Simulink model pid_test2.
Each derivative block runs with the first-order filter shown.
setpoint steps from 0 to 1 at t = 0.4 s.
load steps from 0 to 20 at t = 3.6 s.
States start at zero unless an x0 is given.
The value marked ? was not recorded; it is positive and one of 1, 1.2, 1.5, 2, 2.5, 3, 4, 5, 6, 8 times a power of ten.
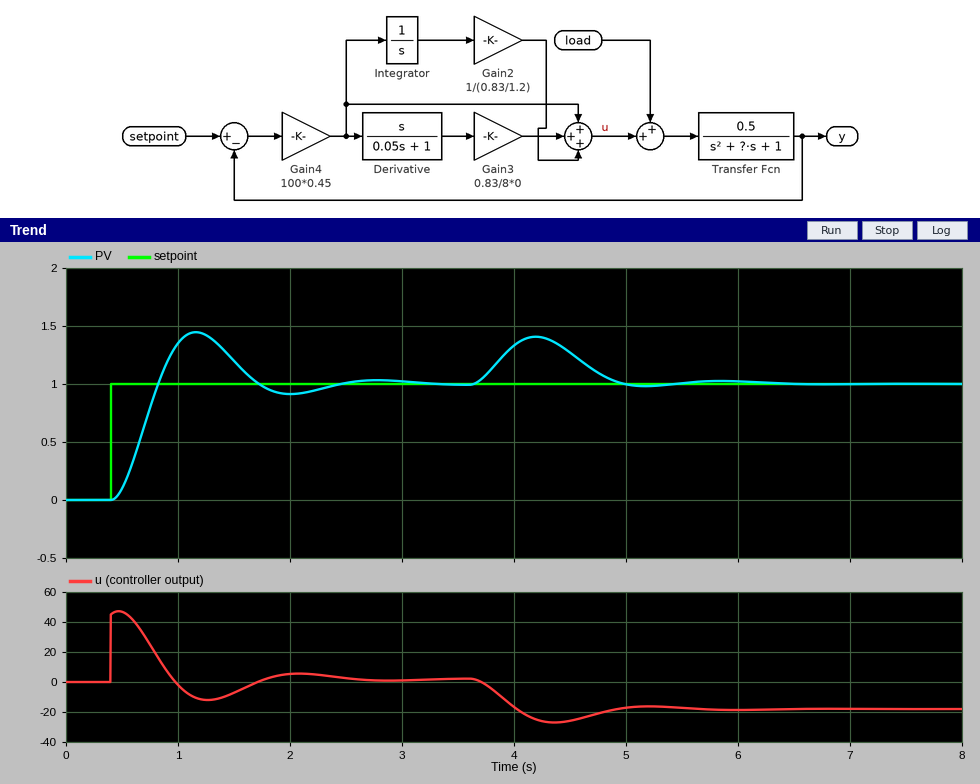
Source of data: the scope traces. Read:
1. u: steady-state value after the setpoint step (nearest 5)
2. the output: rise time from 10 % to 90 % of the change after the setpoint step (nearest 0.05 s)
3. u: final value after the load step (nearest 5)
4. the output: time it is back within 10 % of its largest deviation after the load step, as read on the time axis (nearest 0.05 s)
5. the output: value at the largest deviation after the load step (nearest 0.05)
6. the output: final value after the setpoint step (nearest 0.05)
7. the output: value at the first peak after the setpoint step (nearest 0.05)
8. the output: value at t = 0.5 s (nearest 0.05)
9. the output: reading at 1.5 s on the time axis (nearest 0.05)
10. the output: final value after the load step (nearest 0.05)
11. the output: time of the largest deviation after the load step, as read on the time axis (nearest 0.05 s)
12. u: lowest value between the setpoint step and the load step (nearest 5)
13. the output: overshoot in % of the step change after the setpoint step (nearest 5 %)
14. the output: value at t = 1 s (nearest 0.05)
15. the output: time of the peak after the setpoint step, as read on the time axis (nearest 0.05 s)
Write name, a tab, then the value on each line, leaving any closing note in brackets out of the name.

u: steady-state value after the setpoint step	0
the output: rise time from 10 % to 90 % of the change after the setpoint step	0.30 s
u: final value after the load step	-20
the output: time it is back within 10 % of its largest deviation after the load step, as read on the time axis	4.85 s
the output: value at the largest deviation after the load step	1.40
the output: final value after the setpoint step	1.00
the output: value at the first peak after the setpoint step	1.45
the output: value at t = 0.5 s	0.10
the output: reading at 1.5 s on the time axis	1.20
the output: final value after the load step	1.00
the output: time of the largest deviation after the load step, as read on the time axis	4.20 s
u: lowest value between the setpoint step and the load step	-10
the output: overshoot in % of the step change after the setpoint step	45 %
the output: value at t = 1 s	1.35
the output: time of the peak after the setpoint step, as read on the time axis	1.15 s
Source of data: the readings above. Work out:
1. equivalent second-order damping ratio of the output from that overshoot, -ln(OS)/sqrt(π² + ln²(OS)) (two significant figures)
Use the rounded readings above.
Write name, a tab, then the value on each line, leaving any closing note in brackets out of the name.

equivalent second-order damping ratio of the output from that overshoot, -ln(OS)/sqrt(π² + ln²(OS))	0.25
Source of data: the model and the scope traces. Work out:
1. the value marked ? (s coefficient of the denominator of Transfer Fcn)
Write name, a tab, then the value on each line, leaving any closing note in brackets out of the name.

the value marked ?	5
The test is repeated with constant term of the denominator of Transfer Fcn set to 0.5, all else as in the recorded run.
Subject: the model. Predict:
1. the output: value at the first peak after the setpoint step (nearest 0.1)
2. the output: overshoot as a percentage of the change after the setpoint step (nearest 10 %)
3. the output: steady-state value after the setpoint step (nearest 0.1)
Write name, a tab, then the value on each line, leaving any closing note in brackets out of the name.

the output: value at the first peak after the setpoint step	1.5
the output: overshoot as a percentage of the change after the setpoint step	50 %
the output: steady-state value after the setpoint step	1.0
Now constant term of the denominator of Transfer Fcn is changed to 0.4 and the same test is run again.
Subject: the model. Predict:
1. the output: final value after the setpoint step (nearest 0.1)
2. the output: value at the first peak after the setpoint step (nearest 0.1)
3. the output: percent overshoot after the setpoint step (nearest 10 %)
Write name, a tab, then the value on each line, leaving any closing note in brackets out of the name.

the output: final value after the setpoint step	1.0
the output: value at the first peak after the setpoint step	1.5
the output: percent overshoot after the setpoint step	50 %
